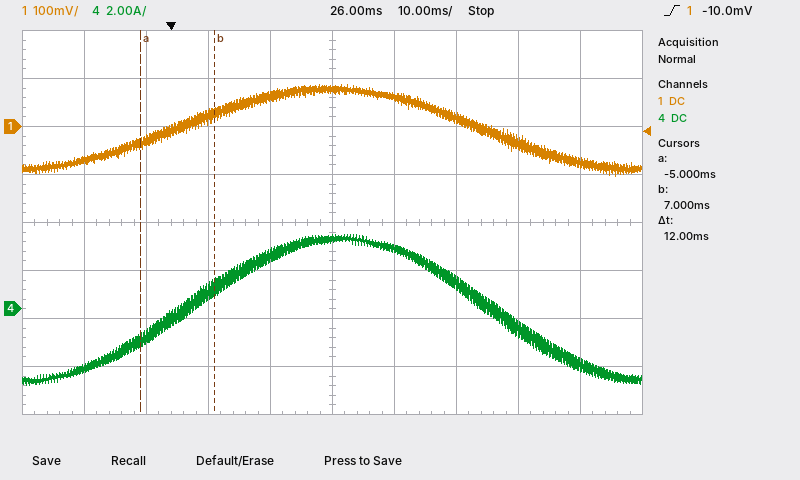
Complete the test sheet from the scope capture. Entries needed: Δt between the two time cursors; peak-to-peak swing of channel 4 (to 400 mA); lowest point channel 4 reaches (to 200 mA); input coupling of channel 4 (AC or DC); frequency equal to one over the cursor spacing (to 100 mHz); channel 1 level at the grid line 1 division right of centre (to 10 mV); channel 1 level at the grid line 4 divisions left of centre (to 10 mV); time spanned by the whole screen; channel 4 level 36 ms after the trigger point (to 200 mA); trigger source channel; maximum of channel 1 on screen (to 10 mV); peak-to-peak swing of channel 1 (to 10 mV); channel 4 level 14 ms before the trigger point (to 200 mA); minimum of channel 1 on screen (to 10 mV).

12 ms
6.4 A
-3.2 A
DC
83.3 Hz
60 mV
-70 mV
100 ms
2.6 A
channel 1
90 mV
190 mV
-2.4 A
-100 mV
